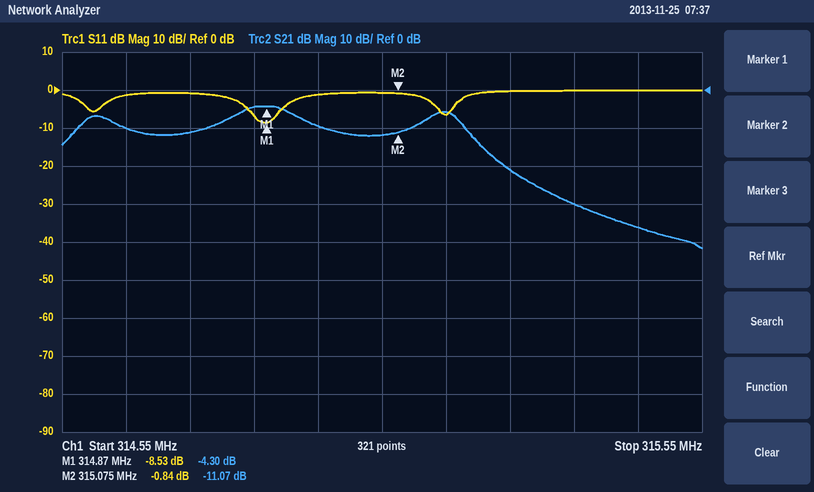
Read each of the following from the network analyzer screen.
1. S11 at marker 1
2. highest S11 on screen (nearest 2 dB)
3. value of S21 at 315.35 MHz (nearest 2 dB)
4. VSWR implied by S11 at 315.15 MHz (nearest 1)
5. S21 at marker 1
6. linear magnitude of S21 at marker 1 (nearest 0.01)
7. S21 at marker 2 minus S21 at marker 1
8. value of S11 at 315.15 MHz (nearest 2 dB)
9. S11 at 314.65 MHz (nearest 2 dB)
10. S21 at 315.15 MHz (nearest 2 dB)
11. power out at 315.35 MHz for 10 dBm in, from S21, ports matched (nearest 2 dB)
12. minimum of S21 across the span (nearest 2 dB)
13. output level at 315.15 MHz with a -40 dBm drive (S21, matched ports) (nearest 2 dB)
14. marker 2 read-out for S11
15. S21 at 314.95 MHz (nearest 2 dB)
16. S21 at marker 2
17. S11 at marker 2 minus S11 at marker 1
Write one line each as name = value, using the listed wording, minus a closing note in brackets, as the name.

S11 at marker 1 = -8.53 dB
highest S11 on screen = 0 dB
value of S21 at 315.35 MHz = -30 dB
VSWR implied by S11 at 315.15 MHz = 3
S21 at marker 1 = -4.30 dB
linear magnitude of S21 at marker 1 = 0.61
S21 at marker 2 minus S21 at marker 1 = -6.77 dB
value of S11 at 315.15 MHz = -6 dB
S11 at 314.65 MHz = -2 dB
S21 at 315.15 MHz = -6 dB
power out at 315.35 MHz for 10 dBm in, from S21, ports matched = -20 dBm
minimum of S21 across the span = -42 dB
output level at 315.15 MHz with a -40 dBm drive (S21, matched ports) = -46 dBm
marker 2 read-out for S11 = -0.84 dB
S21 at 314.95 MHz = -10 dB
S21 at marker 2 = -11.07 dB
S11 at marker 2 minus S11 at marker 1 = 7.69 dB
